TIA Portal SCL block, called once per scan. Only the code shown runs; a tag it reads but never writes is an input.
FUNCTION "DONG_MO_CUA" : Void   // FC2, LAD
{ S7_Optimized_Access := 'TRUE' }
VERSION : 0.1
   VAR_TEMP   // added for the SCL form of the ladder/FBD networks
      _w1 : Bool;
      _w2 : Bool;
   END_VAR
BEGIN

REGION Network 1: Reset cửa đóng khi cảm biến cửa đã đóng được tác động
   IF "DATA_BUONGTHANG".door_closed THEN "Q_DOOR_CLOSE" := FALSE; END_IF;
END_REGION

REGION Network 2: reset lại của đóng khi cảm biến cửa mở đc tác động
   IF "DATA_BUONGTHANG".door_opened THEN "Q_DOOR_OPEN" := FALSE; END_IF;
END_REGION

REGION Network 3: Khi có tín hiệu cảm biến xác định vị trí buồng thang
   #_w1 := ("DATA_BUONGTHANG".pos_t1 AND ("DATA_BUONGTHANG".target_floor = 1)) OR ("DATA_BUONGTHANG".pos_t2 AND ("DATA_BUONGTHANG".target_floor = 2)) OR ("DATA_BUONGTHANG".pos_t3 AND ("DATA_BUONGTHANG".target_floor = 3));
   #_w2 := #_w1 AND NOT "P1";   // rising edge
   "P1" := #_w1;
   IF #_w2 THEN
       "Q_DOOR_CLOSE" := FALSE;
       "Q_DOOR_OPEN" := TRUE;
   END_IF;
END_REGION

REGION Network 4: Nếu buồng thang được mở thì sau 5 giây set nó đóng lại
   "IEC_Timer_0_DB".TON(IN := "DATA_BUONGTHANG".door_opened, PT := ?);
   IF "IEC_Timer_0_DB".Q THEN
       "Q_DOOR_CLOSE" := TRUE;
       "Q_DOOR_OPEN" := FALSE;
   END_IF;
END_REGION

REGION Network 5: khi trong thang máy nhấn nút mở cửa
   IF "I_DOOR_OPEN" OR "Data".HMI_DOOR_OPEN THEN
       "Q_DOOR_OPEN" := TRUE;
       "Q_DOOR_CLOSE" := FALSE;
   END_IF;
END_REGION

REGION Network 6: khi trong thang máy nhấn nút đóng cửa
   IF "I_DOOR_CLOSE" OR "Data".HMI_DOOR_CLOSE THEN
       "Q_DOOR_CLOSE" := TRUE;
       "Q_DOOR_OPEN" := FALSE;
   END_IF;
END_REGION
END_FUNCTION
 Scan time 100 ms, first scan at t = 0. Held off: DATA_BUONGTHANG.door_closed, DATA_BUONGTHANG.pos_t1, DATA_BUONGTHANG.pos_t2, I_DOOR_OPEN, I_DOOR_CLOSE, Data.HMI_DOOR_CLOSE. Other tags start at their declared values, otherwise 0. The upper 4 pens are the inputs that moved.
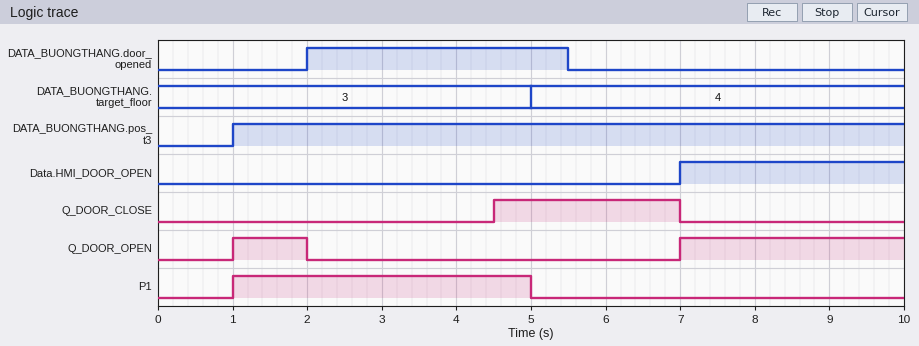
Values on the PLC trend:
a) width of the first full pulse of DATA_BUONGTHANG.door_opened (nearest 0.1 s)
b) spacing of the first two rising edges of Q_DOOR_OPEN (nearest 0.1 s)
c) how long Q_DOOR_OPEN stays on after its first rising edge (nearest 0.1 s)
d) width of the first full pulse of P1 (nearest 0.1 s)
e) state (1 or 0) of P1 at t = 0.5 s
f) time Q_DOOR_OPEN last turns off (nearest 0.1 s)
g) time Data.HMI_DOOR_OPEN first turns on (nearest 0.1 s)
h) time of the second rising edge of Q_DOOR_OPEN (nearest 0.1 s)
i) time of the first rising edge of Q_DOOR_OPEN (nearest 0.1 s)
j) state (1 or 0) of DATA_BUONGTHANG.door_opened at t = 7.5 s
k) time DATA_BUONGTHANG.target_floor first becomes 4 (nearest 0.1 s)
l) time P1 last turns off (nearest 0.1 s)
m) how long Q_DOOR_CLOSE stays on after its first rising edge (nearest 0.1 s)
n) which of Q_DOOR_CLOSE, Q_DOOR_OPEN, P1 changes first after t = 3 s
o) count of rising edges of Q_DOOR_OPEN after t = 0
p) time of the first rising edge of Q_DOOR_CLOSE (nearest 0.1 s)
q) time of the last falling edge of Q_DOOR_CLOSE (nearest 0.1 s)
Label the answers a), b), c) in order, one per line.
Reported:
a) 3.5 s
b) 6.0 s
c) 1.0 s
d) 4.0 s
e) 0
f) 2.0 s
g) 7.0 s
h) 7.0 s
i) 1.0 s
j) 0
k) 5.0 s
l) 5.0 s
m) 2.5 s
n) Q_DOOR_CLOSE
o) 2
p) 4.5 s
q) 7.0 s
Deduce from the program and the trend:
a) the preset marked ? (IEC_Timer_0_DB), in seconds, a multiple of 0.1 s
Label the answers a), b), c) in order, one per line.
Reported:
a) 2.5 s
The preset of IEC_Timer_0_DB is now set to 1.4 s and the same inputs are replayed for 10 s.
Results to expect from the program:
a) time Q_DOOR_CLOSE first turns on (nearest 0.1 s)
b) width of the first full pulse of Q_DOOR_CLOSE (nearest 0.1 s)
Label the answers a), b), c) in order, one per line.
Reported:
a) 3.4 s
b) 3.6 s
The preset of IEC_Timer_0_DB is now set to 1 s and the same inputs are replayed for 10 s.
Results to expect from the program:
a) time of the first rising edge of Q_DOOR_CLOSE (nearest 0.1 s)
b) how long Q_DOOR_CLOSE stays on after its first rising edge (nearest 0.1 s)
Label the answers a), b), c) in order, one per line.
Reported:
a) 3.0 s
b) 4.0 s
